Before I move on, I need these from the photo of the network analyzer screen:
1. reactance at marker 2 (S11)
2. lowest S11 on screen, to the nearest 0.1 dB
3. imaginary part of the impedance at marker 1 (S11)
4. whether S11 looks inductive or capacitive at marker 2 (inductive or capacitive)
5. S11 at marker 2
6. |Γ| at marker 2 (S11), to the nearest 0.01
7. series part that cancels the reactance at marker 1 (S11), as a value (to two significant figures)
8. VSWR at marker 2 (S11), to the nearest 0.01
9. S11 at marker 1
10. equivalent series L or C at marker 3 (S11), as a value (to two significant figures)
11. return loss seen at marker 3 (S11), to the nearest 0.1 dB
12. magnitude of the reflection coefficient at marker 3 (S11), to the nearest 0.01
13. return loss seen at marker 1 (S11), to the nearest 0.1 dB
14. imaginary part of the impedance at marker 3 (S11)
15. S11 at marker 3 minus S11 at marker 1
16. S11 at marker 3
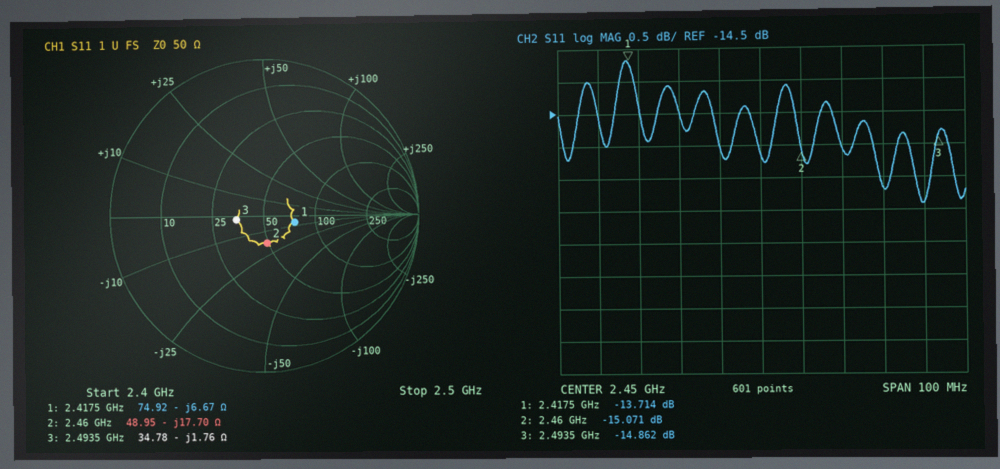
-17.70 Ω
-15.9 dB
-6.67 Ω
capacitive
-15.071 dB
0.18
440 pH
1.43
-13.714 dB
36 pF
14.9 dB
0.18
13.7 dB
-1.76 Ω
-1.148 dB
-14.862 dB
